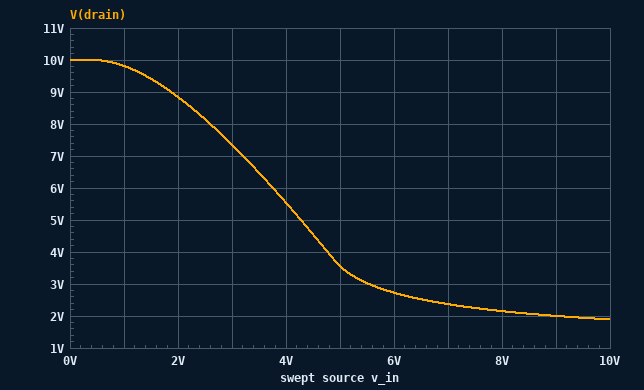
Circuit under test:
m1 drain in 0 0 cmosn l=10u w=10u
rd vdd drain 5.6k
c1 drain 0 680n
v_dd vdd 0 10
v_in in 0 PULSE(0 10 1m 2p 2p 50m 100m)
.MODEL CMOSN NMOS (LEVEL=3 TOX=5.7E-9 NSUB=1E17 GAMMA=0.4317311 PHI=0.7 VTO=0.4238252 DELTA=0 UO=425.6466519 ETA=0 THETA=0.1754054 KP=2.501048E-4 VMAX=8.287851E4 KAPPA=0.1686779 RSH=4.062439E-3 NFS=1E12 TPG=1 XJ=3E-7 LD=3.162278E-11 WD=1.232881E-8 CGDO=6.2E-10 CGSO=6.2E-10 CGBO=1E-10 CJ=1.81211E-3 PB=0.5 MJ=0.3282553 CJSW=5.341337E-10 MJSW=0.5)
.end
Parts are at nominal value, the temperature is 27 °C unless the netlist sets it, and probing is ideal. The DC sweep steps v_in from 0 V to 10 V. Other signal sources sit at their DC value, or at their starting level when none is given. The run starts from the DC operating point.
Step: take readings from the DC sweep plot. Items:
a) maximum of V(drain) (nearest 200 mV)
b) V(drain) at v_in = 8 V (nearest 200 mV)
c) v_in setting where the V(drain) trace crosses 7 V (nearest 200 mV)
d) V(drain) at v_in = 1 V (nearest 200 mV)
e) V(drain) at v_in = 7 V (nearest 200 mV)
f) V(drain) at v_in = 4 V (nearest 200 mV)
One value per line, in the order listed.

10.0 V
2.2 V
3.2 V
9.8 V
2.4 V
5.6 V
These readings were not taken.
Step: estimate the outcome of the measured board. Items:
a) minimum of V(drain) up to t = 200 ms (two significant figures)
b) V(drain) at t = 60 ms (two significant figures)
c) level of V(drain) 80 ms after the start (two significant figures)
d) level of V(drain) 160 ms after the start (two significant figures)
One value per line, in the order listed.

1.9 V
9.2 V
10 V
9.2 V
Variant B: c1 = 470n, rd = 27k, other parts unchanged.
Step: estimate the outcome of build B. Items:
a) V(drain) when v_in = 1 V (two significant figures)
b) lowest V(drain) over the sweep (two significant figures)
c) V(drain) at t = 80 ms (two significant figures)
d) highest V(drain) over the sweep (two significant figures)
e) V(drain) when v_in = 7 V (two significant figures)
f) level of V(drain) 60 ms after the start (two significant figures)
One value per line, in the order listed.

9.1 V
410 mV
9.0 V
10 V
490 mV
5.3 V
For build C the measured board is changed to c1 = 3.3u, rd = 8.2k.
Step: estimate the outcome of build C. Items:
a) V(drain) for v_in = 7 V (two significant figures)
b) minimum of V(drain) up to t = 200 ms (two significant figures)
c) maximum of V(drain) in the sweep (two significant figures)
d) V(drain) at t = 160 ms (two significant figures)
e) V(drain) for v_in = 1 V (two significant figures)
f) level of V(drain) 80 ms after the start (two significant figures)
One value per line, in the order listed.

1.6 V
1.3 V
10 V
3.8 V
9.7 V
7.0 V
